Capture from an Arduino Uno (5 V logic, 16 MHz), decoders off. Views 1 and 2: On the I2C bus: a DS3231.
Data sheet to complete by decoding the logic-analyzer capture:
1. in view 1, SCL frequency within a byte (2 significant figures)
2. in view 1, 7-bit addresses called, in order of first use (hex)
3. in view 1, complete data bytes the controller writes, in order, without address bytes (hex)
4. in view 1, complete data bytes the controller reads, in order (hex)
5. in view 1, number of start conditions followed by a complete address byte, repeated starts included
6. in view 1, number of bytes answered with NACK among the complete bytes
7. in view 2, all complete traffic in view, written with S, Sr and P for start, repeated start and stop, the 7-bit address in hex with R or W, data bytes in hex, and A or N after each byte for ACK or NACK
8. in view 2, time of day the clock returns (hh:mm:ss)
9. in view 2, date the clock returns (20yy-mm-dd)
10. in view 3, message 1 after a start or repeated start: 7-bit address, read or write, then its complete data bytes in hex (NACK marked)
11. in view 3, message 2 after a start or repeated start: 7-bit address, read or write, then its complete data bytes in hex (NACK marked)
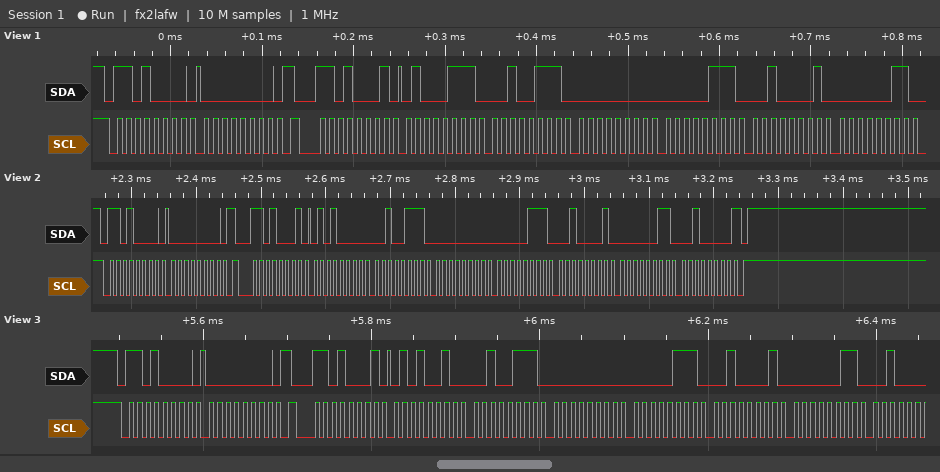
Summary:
100 kHz
0x68
00
47 27 00 07 21 03
2
0
S 68W A 00 A Sr 68R A 50 A 27 A 00 A 07 A 21 A 03 A 20 N P
00:27:50
2020-03-21
0x68 write: 00
0x68 read: 52 27 00 07 21 03
